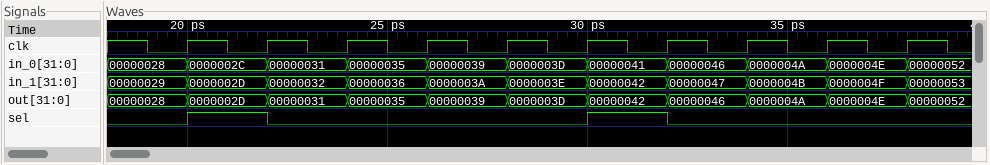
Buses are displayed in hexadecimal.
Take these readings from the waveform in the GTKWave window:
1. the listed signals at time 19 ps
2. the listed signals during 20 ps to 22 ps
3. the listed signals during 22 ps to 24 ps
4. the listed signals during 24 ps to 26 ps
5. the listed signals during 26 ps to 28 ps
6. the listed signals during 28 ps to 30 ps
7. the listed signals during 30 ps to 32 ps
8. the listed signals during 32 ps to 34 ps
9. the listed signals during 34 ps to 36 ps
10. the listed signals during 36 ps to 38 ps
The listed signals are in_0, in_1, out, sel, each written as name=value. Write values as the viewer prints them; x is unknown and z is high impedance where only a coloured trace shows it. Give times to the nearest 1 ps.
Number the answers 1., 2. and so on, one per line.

1. in_0=00000028, in_1=00000029, out=00000028, sel=0
2. in_0=0000002C, in_1=0000002D, out=0000002D, sel=1
3. in_0=00000031, in_1=00000032, out=00000031, sel=0
4. in_0=00000035, in_1=00000036, out=00000035, sel=0
5. in_0=00000039, in_1=0000003A, out=00000039, sel=0
6. in_0=0000003D, in_1=0000003E, out=0000003D, sel=0
7. in_0=00000041, in_1=00000042, out=00000042, sel=1
8. in_0=00000046, in_1=00000047, out=00000046, sel=0
9. in_0=0000004A, in_1=0000004B, out=0000004A, sel=0
10. in_0=0000004E, in_1=0000004F, out=0000004E, sel=0
